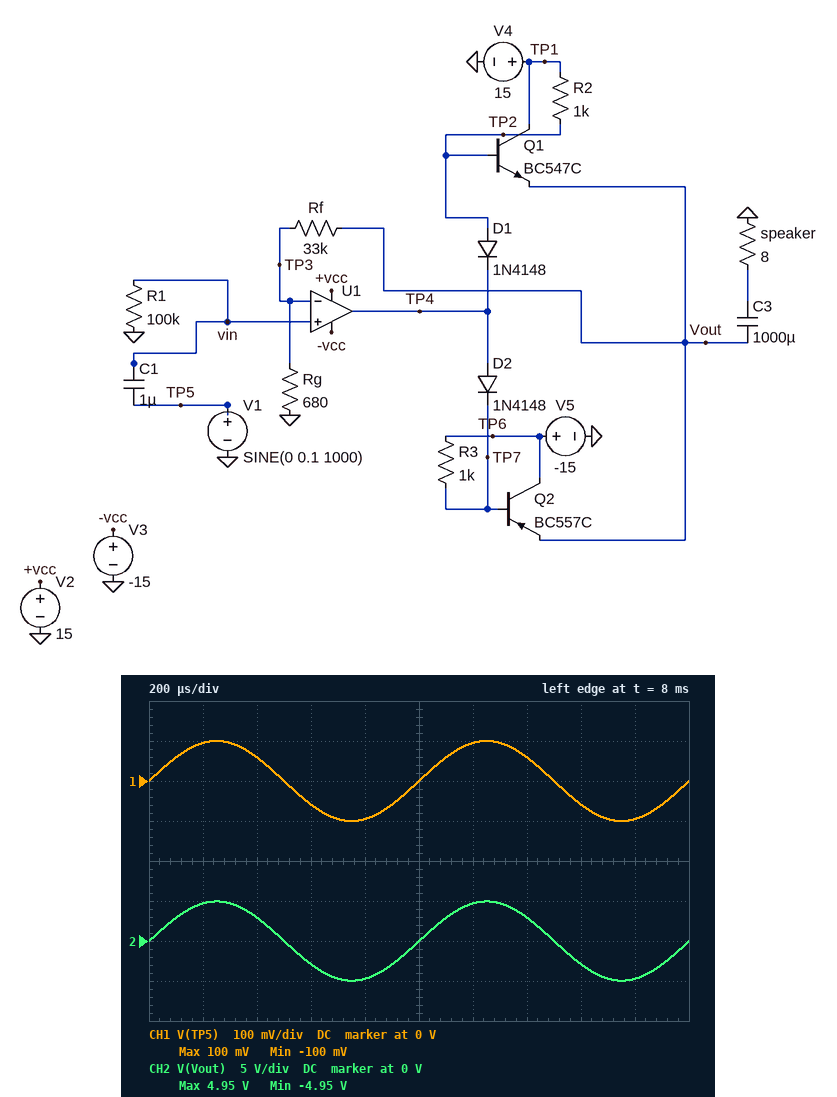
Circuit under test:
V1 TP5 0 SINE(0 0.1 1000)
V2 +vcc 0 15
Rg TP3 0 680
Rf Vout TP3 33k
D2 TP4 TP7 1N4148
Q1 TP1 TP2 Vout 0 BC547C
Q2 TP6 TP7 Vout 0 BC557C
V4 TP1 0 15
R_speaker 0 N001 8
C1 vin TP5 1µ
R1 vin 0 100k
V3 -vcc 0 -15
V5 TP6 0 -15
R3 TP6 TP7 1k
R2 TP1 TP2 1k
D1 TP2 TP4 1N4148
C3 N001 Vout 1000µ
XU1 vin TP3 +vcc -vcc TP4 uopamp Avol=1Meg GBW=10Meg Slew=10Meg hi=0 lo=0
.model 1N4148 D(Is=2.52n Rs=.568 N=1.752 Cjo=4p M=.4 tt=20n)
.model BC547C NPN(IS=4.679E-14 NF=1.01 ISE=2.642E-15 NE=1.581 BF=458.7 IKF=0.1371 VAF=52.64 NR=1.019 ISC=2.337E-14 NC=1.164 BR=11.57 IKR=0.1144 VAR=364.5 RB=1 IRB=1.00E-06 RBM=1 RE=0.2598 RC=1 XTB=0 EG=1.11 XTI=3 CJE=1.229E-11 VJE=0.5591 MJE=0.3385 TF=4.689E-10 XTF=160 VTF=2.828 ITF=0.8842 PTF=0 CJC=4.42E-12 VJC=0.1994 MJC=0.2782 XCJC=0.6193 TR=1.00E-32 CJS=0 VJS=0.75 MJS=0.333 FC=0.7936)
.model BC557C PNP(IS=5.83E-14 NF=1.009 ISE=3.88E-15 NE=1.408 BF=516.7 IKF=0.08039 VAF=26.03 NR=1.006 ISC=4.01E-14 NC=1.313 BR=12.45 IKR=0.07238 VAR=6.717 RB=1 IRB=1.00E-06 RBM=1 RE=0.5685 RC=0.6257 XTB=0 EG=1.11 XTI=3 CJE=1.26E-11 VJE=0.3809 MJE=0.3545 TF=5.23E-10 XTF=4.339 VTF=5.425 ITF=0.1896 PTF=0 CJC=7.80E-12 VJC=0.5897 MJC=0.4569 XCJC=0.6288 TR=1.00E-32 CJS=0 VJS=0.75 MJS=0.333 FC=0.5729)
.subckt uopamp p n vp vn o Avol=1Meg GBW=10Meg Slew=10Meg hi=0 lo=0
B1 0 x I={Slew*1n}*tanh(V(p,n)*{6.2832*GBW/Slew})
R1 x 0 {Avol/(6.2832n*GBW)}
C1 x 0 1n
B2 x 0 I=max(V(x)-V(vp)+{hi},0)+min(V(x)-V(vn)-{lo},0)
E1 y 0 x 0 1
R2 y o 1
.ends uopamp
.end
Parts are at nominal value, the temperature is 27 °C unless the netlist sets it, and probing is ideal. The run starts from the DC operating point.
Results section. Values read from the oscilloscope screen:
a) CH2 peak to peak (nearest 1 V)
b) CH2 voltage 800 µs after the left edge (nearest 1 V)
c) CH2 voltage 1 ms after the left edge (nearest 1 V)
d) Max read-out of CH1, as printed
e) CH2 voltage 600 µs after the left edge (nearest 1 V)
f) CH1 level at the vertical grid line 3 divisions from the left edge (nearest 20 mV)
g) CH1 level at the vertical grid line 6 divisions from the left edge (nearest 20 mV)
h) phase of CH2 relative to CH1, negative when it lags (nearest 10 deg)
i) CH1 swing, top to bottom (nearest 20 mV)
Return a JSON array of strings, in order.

["10 V", "-5 V", "0 V", "100 mV", "-3 V", "-60 mV", "100 mV", "0 deg", "200 mV"]
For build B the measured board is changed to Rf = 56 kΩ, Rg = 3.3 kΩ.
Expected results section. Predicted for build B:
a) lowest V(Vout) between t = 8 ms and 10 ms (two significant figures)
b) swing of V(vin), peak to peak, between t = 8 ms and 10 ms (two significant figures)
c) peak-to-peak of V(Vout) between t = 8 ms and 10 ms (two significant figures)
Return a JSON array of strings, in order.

["-1.8 V", "200 mV", "3.6 V"]
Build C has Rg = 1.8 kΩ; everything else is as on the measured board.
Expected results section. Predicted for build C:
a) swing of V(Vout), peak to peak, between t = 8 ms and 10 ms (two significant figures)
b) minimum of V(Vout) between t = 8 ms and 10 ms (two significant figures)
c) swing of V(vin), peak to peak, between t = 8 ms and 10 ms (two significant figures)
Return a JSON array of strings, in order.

["3.9 V", "-1.9 V", "200 mV"]
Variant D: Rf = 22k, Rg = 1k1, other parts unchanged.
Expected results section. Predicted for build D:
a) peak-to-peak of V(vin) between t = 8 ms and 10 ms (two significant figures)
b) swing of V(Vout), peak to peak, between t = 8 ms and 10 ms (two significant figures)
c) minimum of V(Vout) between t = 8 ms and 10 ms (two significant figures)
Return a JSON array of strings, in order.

["200 mV", "4.2 V", "-2.1 V"]
